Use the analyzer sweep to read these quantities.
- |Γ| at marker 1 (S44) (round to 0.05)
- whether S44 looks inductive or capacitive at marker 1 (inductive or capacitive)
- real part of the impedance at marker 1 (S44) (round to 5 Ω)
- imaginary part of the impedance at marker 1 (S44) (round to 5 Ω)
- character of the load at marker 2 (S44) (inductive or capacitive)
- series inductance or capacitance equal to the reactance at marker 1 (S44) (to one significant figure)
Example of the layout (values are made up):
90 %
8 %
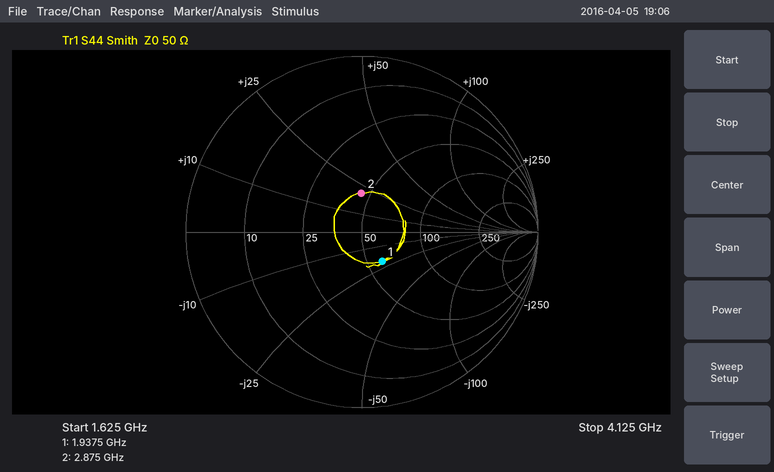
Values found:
0.20
capacitive
60 Ω
-20 Ω
inductive
4 pF
